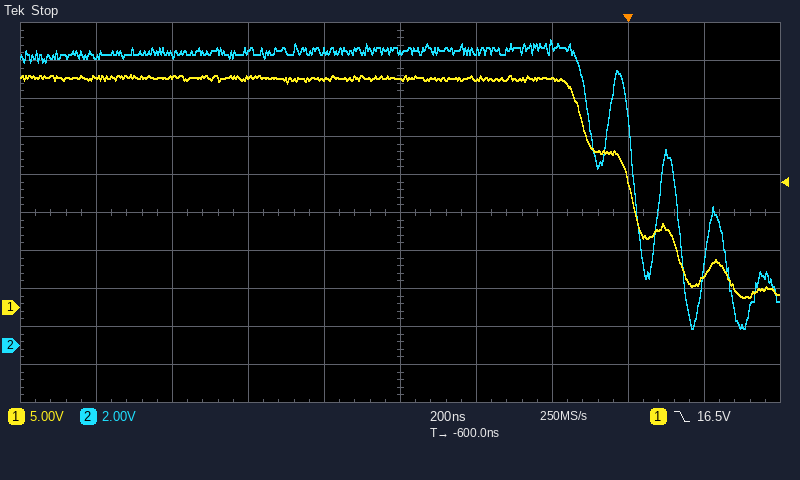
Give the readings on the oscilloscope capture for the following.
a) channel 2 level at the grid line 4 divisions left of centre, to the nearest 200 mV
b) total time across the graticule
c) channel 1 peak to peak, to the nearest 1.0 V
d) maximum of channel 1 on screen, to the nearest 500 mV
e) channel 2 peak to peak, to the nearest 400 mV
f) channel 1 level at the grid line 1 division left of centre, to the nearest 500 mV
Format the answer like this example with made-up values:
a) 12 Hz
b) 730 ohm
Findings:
a) 15.2 V
b) 2 µs
c) 29.0 V
d) 30.5 V
e) 15.2 V
f) 30.0 V
